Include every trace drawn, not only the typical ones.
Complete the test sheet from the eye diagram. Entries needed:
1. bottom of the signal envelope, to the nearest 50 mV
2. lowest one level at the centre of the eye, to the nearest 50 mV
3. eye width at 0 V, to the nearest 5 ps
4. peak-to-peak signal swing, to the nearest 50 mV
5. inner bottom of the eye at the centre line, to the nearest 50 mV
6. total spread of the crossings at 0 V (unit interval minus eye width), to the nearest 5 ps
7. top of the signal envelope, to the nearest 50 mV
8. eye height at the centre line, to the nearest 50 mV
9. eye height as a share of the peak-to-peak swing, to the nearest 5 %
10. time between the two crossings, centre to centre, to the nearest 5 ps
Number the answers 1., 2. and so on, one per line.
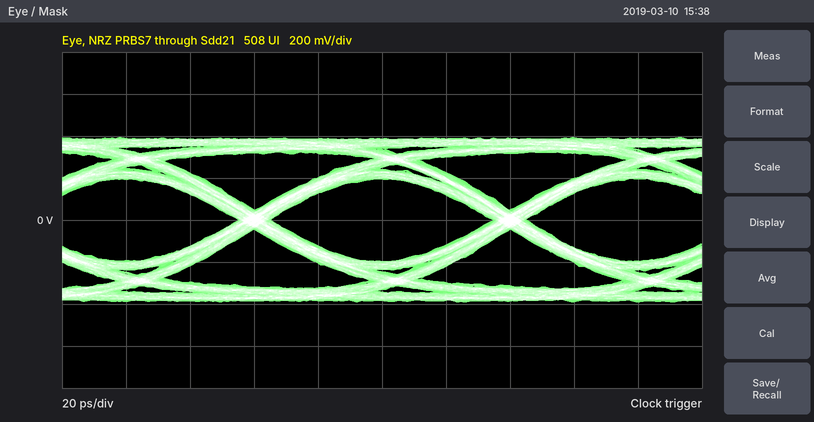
1. -400 mV
2. 200 mV
3. 70 ps
4. 800 mV
5. -200 mV
6. 10 ps
7. 400 mV
8. 400 mV
9. 50 %
10. 80 ps
